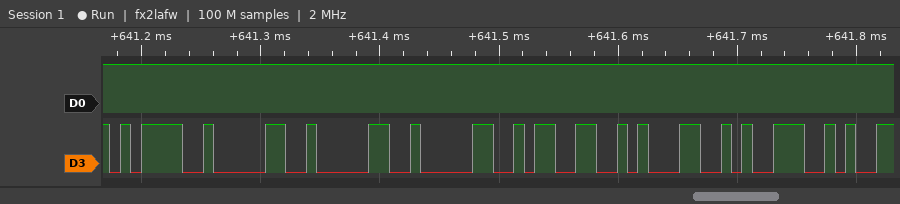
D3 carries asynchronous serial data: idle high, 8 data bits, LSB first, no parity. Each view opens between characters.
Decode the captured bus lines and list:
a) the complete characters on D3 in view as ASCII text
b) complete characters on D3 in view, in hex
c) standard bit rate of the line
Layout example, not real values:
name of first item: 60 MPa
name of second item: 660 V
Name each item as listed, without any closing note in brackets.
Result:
the complete characters on D3 in view as ASCII text: "=000319"
complete characters on D3 in view, in hex: 3D, 30, 30, 30, 33, 31, 39
standard bit rate of the line: 115200 baud
